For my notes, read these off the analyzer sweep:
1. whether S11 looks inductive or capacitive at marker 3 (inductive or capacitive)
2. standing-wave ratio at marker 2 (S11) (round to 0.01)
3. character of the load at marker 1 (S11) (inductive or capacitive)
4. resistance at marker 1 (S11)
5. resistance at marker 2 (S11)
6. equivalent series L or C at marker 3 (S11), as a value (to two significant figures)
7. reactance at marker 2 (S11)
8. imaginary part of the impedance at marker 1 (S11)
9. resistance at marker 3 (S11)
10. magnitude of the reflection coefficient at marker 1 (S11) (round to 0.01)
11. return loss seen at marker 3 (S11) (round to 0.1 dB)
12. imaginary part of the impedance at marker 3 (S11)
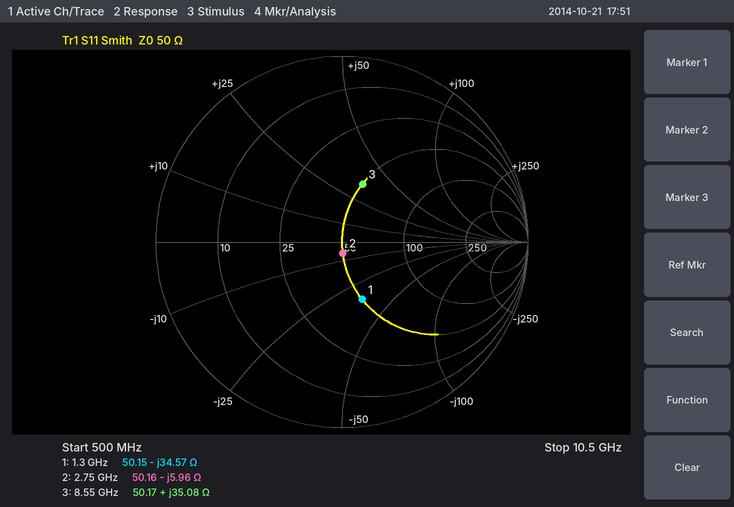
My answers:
inductive
1.13
capacitive
50.15 Ω
50.16 Ω
650 pH
-5.96 Ω
-34.57 Ω
50.17 Ω
0.33
9.6 dB
+35.08 Ω
